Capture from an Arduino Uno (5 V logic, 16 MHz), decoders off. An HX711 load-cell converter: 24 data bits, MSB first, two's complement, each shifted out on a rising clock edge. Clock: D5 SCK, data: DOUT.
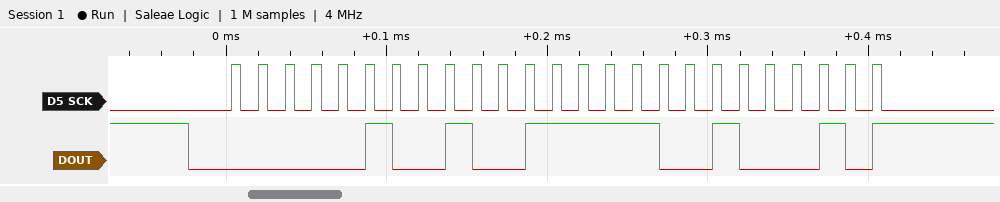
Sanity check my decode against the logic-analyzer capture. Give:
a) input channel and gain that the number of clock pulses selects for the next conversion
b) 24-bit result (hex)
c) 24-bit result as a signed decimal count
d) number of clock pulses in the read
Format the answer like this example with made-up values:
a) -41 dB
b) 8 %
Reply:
a) channel A, gain 128
b) 0x049F22
c) 302882
d) 25
